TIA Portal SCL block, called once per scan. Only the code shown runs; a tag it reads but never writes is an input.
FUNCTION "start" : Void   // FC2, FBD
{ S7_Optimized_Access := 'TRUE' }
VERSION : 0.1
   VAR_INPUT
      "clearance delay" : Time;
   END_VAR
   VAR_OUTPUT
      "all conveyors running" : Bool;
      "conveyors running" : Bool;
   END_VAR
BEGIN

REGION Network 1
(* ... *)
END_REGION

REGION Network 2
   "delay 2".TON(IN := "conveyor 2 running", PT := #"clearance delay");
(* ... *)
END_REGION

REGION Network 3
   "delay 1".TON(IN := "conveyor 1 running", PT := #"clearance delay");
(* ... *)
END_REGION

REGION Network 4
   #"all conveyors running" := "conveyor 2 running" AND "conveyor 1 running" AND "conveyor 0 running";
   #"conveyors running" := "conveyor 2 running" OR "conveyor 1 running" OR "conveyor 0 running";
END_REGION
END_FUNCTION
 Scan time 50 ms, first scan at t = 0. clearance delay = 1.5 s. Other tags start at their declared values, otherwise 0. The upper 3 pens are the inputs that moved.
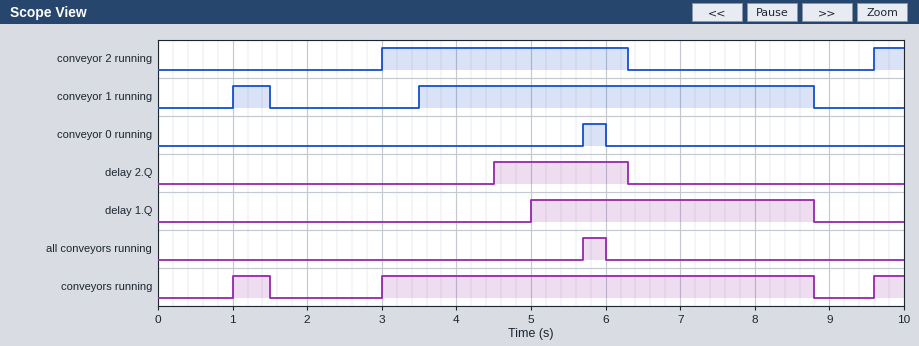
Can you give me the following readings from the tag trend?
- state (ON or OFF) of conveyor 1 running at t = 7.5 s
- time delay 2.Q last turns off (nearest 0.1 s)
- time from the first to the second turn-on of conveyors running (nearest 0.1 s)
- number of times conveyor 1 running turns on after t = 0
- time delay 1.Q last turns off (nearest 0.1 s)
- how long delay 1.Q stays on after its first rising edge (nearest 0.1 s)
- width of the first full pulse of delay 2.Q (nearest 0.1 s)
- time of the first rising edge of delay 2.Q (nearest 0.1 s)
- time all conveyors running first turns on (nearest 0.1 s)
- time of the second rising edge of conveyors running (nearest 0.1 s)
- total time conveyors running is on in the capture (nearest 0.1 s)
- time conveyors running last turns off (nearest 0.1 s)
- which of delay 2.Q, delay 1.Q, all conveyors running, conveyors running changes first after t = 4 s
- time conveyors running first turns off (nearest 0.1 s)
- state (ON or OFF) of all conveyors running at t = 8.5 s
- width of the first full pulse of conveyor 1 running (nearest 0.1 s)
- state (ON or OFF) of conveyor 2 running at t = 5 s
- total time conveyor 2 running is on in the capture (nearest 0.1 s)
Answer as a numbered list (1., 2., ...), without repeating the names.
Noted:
1. ON
2. 6.3 s
3. 2.0 s
4. 2
5. 8.8 s
6. 3.8 s
7. 1.8 s
8. 4.5 s
9. 5.7 s
10. 3.0 s
11. 6.7 s
12. 8.8 s
13. delay 2.Q
14. 1.5 s
15. OFF
16. 0.5 s
17. ON
18. 3.7 s
